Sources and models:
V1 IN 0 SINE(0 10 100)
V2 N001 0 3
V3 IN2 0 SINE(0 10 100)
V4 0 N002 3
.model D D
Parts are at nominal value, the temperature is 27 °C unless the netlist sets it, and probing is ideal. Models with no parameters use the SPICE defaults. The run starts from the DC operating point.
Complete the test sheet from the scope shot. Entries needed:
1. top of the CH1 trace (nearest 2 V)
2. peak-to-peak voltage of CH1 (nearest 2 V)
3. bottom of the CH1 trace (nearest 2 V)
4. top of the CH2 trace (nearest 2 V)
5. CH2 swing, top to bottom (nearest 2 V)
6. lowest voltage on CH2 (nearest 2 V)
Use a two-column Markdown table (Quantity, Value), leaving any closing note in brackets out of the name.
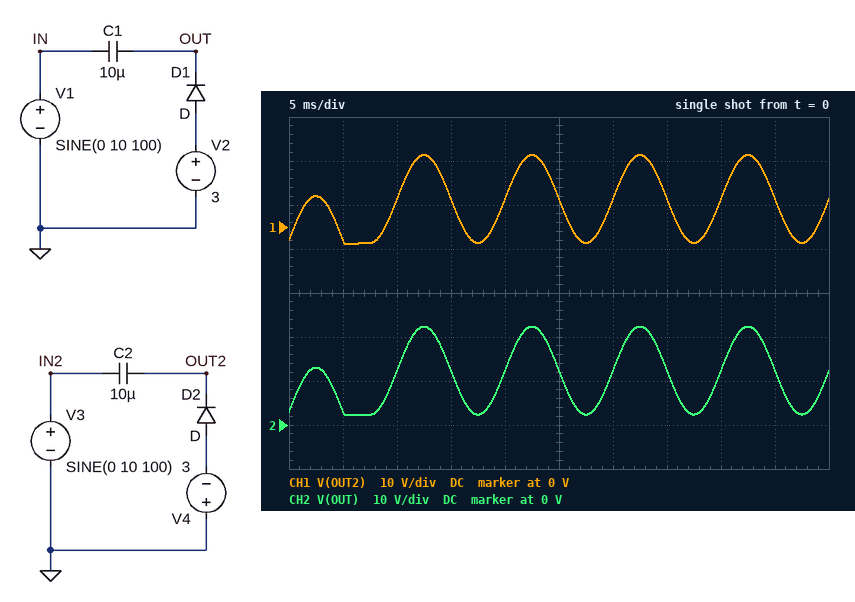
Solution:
| Quantity | Value |
|---|---|
| top of the CH1 trace | 16 V |
| peak-to-peak voltage of CH1 | 20 V |
| bottom of the CH1 trace | -4 V |
| top of the CH2 trace | 22 V |
| CH2 swing, top to bottom | 20 V |
| lowest voltage on CH2 | 2 V |
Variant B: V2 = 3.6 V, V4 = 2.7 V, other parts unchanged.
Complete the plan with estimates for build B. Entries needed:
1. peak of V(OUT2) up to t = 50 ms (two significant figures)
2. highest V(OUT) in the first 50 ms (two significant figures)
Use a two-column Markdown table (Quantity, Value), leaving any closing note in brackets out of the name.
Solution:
| Quantity | Value |
|---|---|
| peak of V(OUT2) up to t = 50 ms | 17 V |
| highest V(OUT) in the first 50 ms | 23 V |
